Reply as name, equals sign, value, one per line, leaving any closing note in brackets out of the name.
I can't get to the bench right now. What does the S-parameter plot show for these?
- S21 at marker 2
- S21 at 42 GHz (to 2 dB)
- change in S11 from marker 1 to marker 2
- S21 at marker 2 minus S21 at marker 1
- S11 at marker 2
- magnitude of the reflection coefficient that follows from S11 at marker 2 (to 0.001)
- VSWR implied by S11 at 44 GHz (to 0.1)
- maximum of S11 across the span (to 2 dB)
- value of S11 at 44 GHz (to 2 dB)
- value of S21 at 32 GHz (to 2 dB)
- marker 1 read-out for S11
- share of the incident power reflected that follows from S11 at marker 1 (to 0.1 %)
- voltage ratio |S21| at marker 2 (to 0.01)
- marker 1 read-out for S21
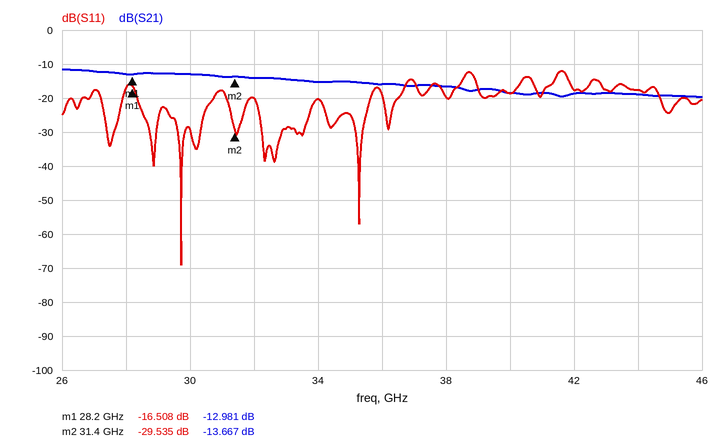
S21 at marker 2 = -13.667 dB
S21 at 42 GHz = -18 dB
change in S11 from marker 1 to marker 2 = -13.027 dB
S21 at marker 2 minus S21 at marker 1 = -0.686 dB
S11 at marker 2 = -29.535 dB
magnitude of the reflection coefficient that follows from S11 at marker 2 = 0.033
VSWR implied by S11 at 44 GHz = 1.3
maximum of S11 across the span = -12 dB
value of S11 at 44 GHz = -18 dB
value of S21 at 32 GHz = -14 dB
marker 1 read-out for S11 = -16.508 dB
share of the incident power reflected that follows from S11 at marker 1 = 2.2 %
voltage ratio |S21| at marker 2 = 0.21
marker 1 read-out for S21 = -12.981 dB
